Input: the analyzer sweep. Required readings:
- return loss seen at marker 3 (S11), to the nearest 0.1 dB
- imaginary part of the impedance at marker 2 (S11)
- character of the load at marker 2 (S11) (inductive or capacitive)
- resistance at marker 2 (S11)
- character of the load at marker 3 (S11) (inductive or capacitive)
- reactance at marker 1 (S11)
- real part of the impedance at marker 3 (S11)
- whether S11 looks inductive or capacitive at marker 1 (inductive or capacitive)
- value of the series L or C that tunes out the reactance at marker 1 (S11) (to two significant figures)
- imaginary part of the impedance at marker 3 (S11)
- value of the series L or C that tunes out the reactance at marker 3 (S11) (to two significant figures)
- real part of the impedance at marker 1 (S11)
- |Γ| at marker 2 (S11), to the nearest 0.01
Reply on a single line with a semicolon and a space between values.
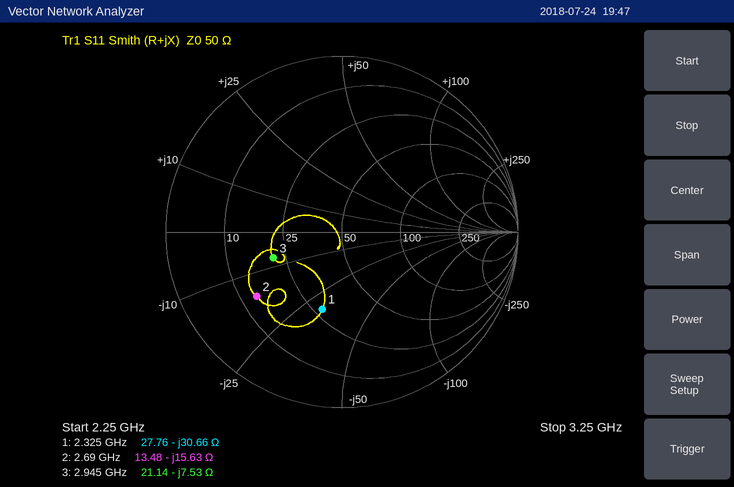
7.6 dB; -15.63 Ω; capacitive; 13.48 Ω; capacitive; -30.66 Ω; 21.14 Ω; capacitive; 2.1 nH; -7.53 Ω; 410 pH; 27.76 Ω; 0.61
